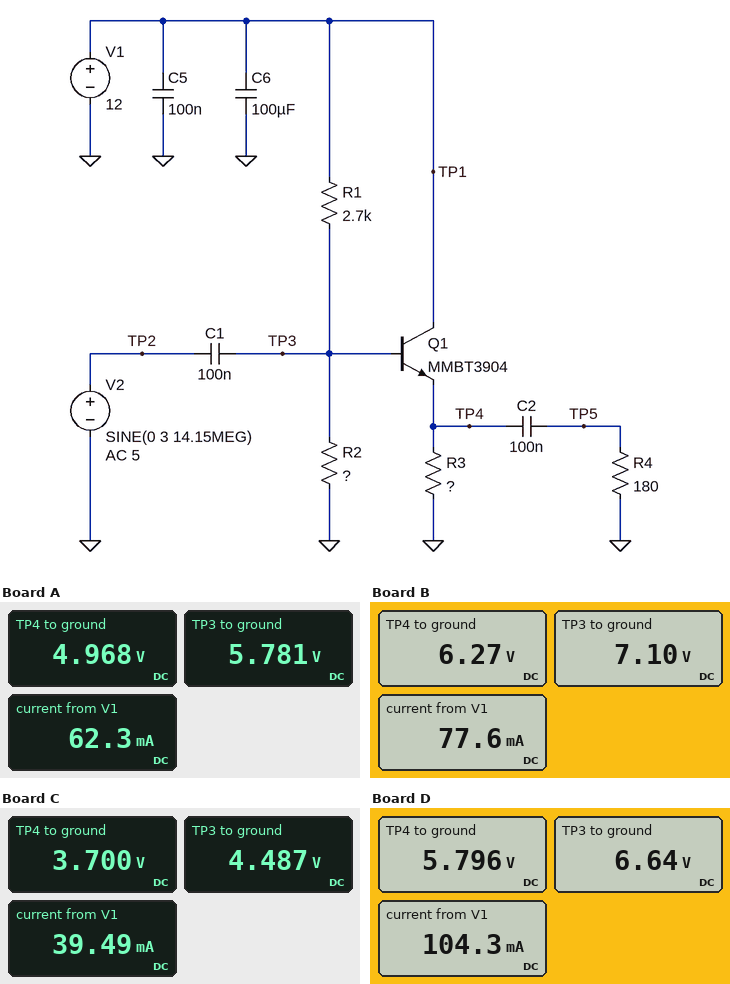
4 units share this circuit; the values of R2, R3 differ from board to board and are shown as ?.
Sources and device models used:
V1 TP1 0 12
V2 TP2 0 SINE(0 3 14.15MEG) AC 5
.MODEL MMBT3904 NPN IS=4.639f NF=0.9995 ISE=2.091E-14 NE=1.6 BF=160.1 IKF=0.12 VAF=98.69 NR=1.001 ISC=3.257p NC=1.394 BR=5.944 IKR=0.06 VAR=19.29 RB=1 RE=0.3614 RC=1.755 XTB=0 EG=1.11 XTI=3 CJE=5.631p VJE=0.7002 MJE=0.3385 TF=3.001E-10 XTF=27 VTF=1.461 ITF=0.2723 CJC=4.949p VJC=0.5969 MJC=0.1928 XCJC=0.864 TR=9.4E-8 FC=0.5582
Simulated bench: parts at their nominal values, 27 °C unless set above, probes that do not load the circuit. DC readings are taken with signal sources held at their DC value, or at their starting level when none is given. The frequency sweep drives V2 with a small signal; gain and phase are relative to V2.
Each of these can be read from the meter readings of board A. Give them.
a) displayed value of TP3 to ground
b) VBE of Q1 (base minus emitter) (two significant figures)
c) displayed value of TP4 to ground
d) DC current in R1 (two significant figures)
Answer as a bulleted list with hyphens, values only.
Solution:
- 5.781 V
- 810 mV
- 4.968 V
- 2.3 mA
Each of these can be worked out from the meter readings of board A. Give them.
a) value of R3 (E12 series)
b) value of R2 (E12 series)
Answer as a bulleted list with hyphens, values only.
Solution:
- 82 Ω
- 3.3 kΩ
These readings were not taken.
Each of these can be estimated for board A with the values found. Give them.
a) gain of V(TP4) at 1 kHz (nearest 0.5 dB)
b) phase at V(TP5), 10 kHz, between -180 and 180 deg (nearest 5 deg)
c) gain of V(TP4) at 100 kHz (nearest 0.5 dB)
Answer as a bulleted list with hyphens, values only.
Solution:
- -4.5 dB
- 50 deg
- 0 dB
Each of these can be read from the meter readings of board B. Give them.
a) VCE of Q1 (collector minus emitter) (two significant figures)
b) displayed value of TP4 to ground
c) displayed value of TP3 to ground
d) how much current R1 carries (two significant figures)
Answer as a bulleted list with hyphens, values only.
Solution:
- 5.7 V
- 6.27 V
- 7.10 V
- 1.8 mA
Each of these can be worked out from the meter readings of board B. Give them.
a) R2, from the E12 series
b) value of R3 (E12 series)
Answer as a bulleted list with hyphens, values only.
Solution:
- 6.8 kΩ
- 82 Ω
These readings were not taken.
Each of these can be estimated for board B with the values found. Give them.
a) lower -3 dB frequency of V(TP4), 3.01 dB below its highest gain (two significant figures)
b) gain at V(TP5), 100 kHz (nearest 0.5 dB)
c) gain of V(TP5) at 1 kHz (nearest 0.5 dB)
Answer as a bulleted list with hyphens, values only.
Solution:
- 1.1 kHz
- 0 dB
- -22.5 dB
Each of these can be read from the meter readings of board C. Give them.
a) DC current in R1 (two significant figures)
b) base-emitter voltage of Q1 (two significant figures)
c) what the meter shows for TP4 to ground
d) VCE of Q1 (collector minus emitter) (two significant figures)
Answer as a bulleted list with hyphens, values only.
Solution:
- 2.8 mA
- 790 mV
- 3.700 V
- 8.3 V
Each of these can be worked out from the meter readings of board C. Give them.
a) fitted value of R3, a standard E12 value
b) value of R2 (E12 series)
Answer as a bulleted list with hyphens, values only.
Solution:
- 100 Ω
- 1.8 kΩ
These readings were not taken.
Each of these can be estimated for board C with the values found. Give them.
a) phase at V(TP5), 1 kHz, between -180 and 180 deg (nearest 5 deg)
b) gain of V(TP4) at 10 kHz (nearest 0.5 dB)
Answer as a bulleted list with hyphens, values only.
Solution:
- 140 deg
- -0.5 dB
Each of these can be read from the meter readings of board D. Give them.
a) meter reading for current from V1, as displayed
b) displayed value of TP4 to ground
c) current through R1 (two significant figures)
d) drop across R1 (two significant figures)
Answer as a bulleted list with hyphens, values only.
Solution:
- 104.3 mA
- 5.796 V
- 2.0 mA
- 5.4 V
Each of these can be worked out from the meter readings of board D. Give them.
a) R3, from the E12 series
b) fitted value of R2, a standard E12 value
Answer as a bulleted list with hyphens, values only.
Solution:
- 56 Ω
- 8.2 kΩ
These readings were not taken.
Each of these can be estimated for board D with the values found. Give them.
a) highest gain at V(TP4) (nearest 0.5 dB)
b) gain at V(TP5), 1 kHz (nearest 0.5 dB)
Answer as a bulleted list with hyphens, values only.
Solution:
- 0 dB
- -23.5 dB
